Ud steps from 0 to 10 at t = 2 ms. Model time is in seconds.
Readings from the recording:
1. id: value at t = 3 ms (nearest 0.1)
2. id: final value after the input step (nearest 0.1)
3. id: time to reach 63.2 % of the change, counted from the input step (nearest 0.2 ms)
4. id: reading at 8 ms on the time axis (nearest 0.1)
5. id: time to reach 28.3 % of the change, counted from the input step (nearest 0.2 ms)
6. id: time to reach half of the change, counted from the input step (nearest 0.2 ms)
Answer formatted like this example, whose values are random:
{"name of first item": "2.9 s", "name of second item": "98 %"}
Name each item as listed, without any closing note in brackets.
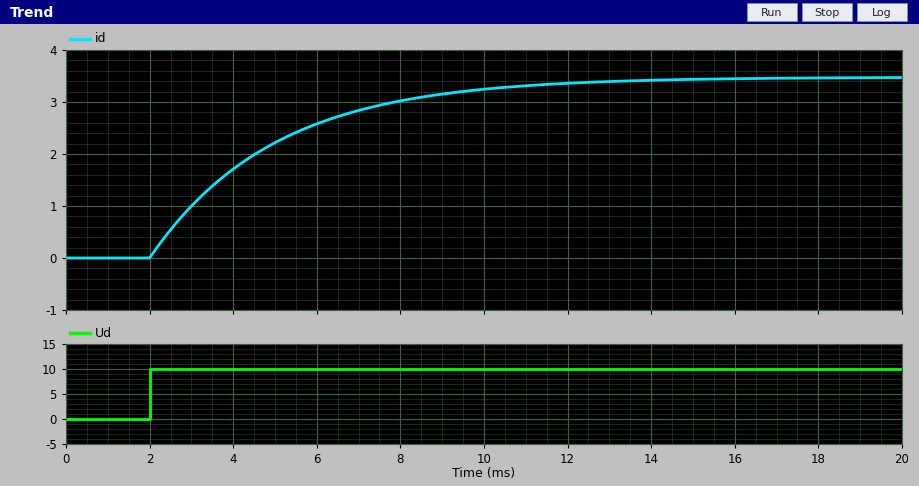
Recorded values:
{"id: value at t = 3 ms": "1.0", "id: final value after the input step": "3.5", "id: time to reach 63.2 % of the change, counted from the input step": "3.0 ms", "id: reading at 8 ms on the time axis": "3.0", "id: time to reach 28.3 % of the change, counted from the input step": "1.0 ms", "id: time to reach half of the change, counted from the input step": "2.0 ms"}
